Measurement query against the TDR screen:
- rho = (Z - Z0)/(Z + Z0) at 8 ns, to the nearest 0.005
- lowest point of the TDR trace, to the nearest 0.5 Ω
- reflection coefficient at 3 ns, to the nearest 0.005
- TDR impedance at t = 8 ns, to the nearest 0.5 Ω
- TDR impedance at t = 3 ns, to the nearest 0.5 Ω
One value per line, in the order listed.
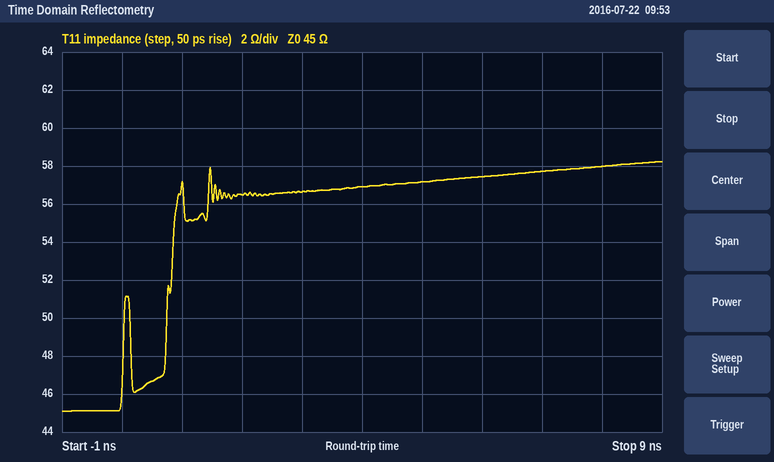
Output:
+0.125
45.0 Ω
+0.115
58.0 Ω
56.5 Ω
